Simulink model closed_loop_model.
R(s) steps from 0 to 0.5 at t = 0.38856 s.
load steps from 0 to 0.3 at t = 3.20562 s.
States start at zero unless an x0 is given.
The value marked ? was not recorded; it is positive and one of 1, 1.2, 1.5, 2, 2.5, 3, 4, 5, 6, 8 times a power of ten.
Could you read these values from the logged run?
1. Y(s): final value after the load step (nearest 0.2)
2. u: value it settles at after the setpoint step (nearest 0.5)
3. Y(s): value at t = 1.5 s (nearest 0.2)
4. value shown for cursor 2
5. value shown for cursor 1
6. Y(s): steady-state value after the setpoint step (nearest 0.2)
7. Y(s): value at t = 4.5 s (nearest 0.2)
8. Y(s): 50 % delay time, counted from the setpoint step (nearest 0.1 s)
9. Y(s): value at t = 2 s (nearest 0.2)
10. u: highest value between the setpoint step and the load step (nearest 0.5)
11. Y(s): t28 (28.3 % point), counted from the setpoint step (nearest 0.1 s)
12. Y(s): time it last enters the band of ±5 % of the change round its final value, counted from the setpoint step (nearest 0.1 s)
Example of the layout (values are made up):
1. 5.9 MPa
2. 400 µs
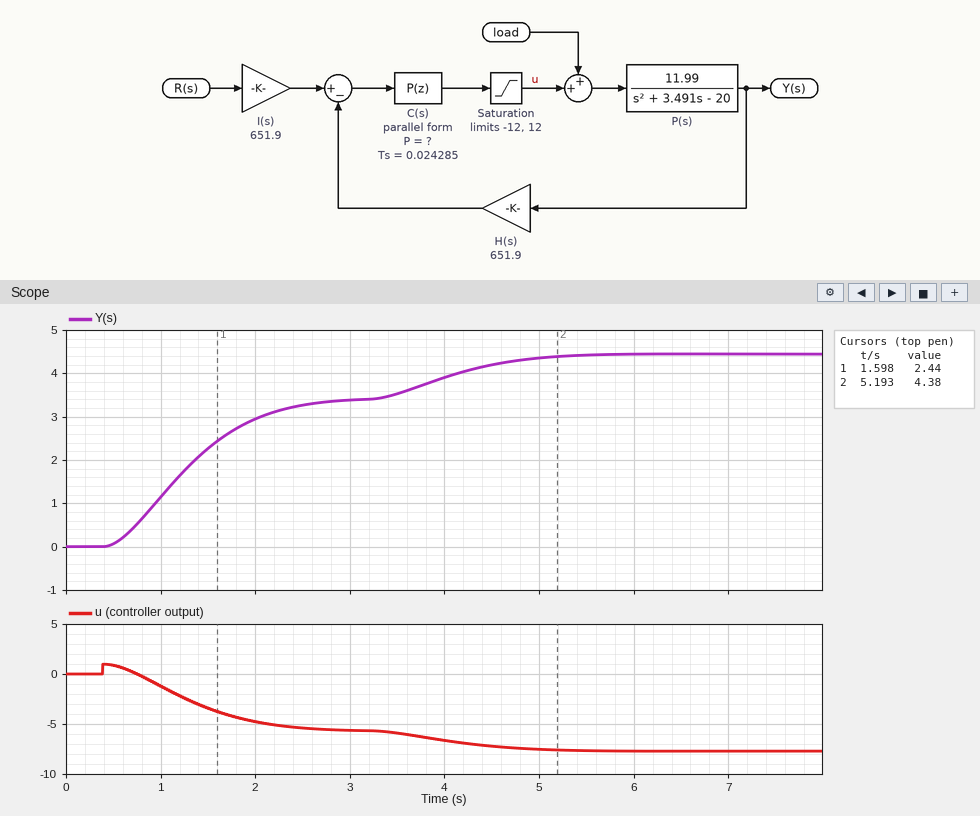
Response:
1. 4.4
2. -5.5
3. 2.2
4. 4.38
5. 2.44
6. 3.4
7. 4.2
8. 0.8 s
9. 3.0
10. 1.0
11. 0.5 s
12. 2.0 s
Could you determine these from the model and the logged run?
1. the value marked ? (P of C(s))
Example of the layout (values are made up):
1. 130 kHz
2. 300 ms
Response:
1. 0.003
